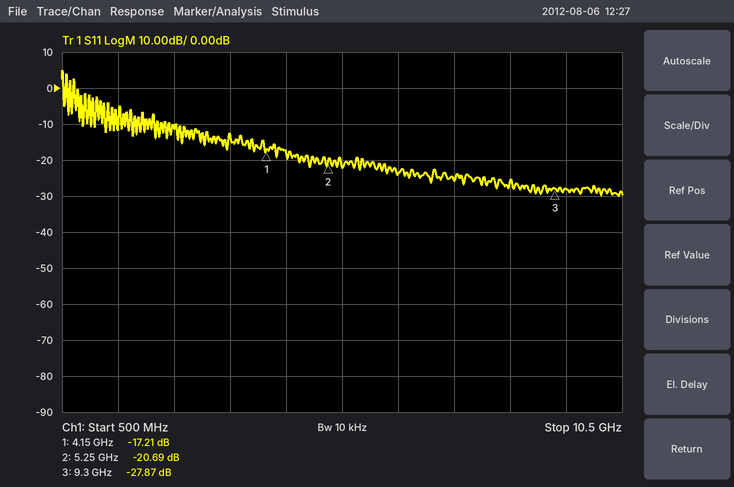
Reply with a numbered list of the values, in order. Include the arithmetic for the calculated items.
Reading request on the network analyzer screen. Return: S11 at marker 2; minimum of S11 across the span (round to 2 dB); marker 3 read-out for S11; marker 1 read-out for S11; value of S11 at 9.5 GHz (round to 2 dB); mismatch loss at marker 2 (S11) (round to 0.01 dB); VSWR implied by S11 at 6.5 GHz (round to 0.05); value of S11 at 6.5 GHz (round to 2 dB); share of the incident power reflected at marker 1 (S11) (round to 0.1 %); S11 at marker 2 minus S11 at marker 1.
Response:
1. -20.69 dB
2. -30 dB
3. -27.87 dB
4. -17.21 dB
5. -28 dB
6. −10 log10(1 − 10^(-20.69/10)) ≈ 0.04 dB
7. |Γ| = 10^(-24/20) = 0.0631; VSWR = (1 + 0.0631)/(1 − 0.0631) ≈ 1.13, so 1.15 to the nearest 0.05
8. -24 dB
9. 10^(-17.21/10) ≈ 1.9 %
10. -20.69 − (-17.21) = -3.48 dB
